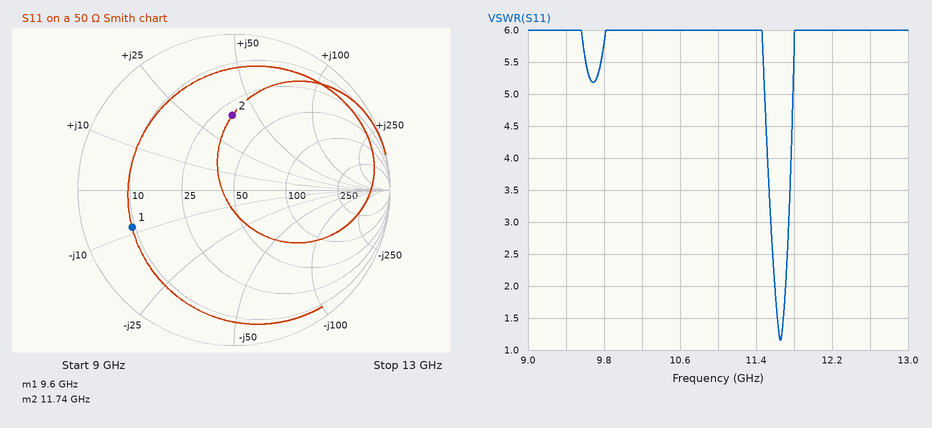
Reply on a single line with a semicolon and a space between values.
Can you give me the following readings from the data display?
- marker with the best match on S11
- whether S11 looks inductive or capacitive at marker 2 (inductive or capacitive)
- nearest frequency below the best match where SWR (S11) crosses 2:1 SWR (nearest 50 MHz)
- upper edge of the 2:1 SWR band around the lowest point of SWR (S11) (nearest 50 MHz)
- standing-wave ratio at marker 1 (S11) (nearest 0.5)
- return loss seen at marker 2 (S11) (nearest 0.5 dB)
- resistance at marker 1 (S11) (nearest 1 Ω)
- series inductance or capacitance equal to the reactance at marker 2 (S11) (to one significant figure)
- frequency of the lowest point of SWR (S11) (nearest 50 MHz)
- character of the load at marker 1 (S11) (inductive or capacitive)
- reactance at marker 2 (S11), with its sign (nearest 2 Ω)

marker 2; inductive; 11.60 GHz; 11.70 GHz; 5.5; 6.5 dB; 9 Ω; 500 pH; 11.65 GHz; capacitive; +38 Ω
